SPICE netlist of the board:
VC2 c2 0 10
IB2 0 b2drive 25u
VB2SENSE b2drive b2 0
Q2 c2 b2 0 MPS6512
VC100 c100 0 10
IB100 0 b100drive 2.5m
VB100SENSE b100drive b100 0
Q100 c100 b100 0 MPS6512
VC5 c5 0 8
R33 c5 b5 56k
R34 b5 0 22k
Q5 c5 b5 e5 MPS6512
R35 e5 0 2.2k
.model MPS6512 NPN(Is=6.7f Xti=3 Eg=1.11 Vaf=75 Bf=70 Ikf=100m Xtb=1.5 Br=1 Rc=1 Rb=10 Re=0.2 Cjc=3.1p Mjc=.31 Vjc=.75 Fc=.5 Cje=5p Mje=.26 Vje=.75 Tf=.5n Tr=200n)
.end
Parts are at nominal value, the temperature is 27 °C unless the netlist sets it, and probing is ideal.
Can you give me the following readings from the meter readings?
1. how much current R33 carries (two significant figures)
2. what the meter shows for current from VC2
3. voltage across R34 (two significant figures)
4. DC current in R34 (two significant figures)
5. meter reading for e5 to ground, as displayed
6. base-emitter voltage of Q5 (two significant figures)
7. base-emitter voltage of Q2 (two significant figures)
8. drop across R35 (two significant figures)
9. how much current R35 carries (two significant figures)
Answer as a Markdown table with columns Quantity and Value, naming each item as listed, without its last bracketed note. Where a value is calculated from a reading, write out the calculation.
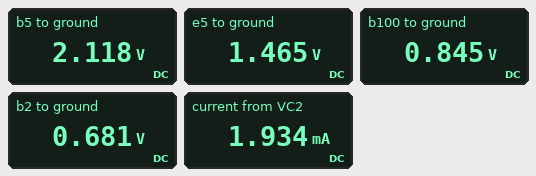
| Quantity | Value |
|---|---|
| how much current R33 carries | (8 V - 2.118 V) / 56 kΩ = 110 µA |
| what the meter shows for current from VC2 | 1.934 mA |
| voltage across R34 | 2.118 V = 2.1 V |
| DC current in R34 | (2.118 V) / 22 kΩ = 96 µA |
| meter reading for e5 to ground, as displayed | 1.465 V |
| base-emitter voltage of Q5 | 2.118 V - 1.465 V = 650 mV |
| base-emitter voltage of Q2 | 681 mV = 680 mV |
| drop across R35 | 1.465 V = 1.5 V |
| how much current R35 carries | (1.465 V) / 2.2 kΩ = 670 µA |
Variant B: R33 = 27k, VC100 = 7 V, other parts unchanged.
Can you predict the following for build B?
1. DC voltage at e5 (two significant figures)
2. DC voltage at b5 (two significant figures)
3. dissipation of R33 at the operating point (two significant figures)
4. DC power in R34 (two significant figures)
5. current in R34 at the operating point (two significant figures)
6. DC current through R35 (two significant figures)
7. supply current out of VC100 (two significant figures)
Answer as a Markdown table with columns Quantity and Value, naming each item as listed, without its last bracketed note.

| Quantity | Value |
|---|---|
| DC voltage at e5 | 2.7 V |
| DC voltage at b5 | 3.4 V |
| dissipation of R33 at the operating point | 790 µW |
| DC power in R34 | 520 µW |
| current in R34 at the operating point | 150 µA |
| DC current through R35 | 1.2 mA |
| supply current out of VC100 | 99 mA |
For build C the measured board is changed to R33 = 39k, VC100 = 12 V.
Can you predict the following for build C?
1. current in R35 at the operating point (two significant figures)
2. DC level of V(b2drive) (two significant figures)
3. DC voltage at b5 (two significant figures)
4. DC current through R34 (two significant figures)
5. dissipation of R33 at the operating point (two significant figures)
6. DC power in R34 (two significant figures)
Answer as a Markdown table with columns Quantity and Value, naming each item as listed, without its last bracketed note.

| Quantity | Value |
|---|---|
| current in R35 at the operating point | 930 µA |
| DC level of V(b2drive) | 680 mV |
| DC voltage at b5 | 2.7 V |
| DC current through R34 | 120 µA |
| dissipation of R33 at the operating point | 720 µW |
| DC power in R34 | 330 µW |
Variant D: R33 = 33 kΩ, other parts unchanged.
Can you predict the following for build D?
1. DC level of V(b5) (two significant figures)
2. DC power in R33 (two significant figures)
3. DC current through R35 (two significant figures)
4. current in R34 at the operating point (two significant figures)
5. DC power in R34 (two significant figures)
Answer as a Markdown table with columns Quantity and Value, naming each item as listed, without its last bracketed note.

| Quantity | Value |
|---|---|
| DC level of V(b5) | 3.0 V |
| DC power in R33 | 750 µW |
| DC current through R35 | 1.1 mA |
| current in R34 at the operating point | 140 µA |
| DC power in R34 | 410 µW |
